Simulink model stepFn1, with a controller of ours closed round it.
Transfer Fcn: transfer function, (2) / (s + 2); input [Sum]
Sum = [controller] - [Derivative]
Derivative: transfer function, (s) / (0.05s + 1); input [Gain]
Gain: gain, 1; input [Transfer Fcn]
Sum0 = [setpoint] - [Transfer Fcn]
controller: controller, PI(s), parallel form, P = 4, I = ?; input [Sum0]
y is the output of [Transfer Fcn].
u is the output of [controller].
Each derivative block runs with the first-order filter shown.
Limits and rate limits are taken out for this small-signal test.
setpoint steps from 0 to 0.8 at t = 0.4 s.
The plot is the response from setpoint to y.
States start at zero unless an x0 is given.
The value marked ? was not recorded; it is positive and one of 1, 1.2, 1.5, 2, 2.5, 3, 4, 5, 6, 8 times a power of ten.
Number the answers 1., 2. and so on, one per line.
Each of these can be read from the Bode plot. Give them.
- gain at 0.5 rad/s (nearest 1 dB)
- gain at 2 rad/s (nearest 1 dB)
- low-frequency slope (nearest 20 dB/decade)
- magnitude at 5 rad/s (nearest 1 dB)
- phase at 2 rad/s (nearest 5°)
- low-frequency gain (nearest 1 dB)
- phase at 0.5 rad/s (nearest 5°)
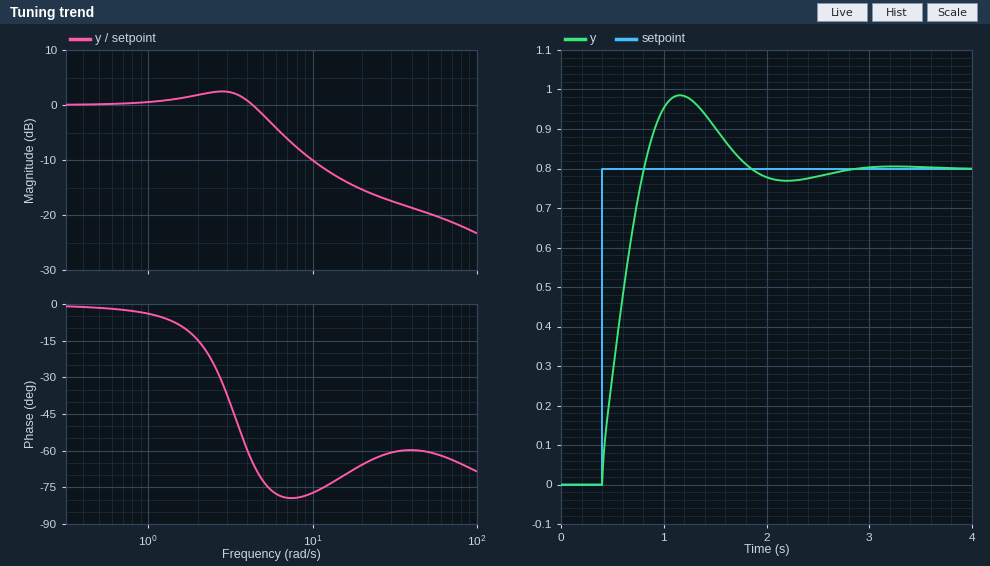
1. 0 dB
2. 2 dB
3. 0 dB/decade
4. -2 dB
5. -15°
6. 0 dB
7. 0°
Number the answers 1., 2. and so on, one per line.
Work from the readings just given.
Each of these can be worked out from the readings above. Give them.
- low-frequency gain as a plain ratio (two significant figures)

1. 1.0
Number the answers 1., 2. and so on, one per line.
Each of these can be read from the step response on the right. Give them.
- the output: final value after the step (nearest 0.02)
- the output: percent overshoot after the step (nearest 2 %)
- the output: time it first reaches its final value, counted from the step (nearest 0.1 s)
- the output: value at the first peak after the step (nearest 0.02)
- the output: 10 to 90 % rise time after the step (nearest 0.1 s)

1. 0.80
2. 24 %
3. 0.4 s
4. 0.98
5. 0.3 s
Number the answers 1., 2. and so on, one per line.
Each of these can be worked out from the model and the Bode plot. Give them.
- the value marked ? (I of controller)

1. 20
